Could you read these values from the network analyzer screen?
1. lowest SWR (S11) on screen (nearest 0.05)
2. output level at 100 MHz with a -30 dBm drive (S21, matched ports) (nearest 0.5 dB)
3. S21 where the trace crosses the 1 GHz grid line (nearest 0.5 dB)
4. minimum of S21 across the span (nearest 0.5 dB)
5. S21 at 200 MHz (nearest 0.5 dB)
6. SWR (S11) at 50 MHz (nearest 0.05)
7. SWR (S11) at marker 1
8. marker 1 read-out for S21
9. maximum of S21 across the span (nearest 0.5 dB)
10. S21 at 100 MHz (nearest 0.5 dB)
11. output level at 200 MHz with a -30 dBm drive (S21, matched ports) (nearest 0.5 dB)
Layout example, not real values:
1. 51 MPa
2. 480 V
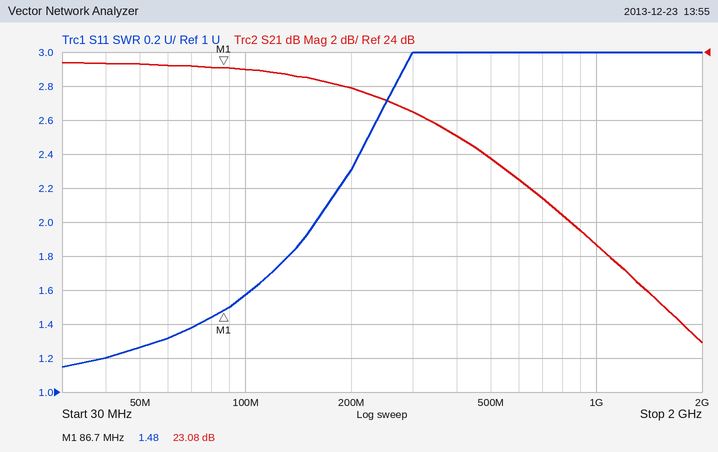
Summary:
1. 1.15
2. -7.0 dBm
3. 12.5 dB
4. 7.0 dB
5. 22.0 dB
6. 1.25
7. 1.48
8. 23.08 dB
9. 23.5 dB
10. 23.0 dB
11. -8.0 dBm
